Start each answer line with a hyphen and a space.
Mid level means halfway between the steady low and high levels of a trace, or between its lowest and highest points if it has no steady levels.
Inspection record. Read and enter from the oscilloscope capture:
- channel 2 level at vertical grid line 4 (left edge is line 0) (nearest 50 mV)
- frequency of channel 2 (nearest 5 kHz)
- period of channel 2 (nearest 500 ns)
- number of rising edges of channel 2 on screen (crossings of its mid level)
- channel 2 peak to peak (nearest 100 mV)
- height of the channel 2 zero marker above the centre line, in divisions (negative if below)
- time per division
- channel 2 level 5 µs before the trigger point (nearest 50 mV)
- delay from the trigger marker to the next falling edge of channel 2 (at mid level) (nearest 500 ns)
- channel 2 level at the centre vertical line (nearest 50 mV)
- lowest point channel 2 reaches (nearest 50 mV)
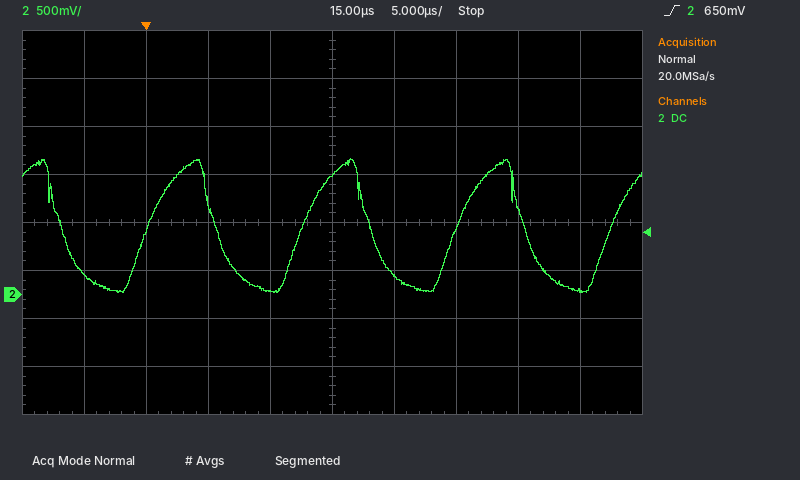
- 50 mV
- 80 kHz
- 12.5 µs
- 4
- 1.40 V
- -1.5 div
- 5 µs
- 200 mV
- 5.5 µs
- 1.25 V
- 0 mV
